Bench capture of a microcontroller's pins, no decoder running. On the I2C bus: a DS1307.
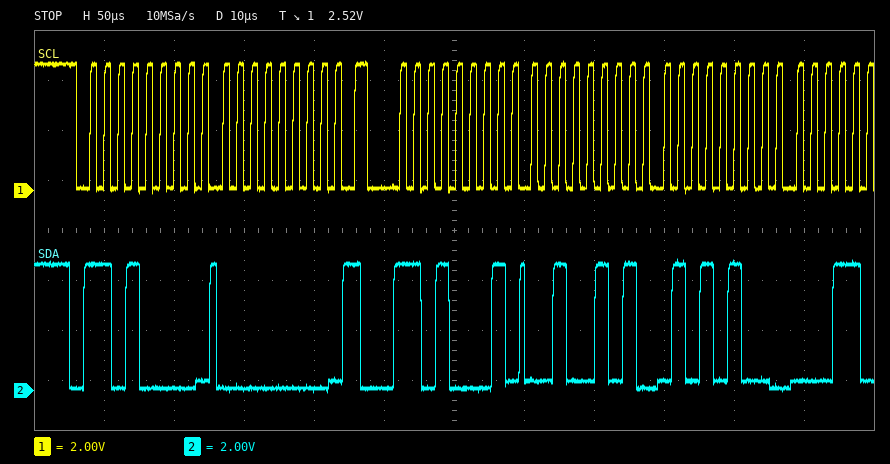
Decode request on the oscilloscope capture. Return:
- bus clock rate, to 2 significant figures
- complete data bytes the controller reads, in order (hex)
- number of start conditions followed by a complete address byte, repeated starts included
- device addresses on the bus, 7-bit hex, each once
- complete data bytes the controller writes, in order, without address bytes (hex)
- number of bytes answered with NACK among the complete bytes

100 kHz
25 54
2
0x68
00
0
